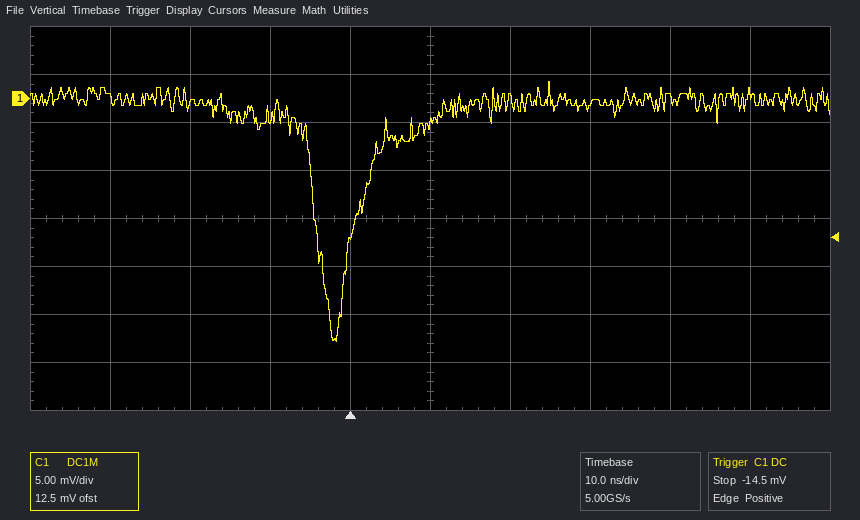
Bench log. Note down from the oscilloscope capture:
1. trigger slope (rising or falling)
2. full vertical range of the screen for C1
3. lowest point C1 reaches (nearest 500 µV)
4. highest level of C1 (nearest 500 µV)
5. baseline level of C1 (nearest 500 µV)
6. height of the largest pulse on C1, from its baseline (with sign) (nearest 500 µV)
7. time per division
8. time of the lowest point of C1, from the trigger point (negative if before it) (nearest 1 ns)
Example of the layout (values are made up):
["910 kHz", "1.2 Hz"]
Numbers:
["rising", "40 mV", "-25.5 mV", "2.0 mV", "-500 µV", "-25.0 mV", "10 ns", "-2 ns"]
